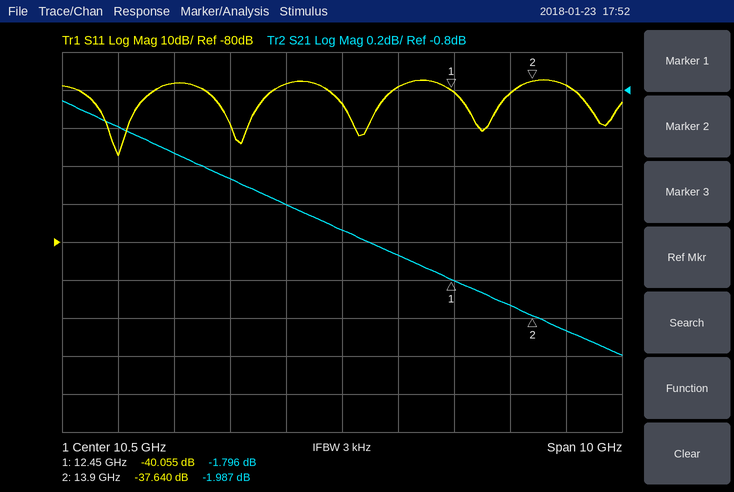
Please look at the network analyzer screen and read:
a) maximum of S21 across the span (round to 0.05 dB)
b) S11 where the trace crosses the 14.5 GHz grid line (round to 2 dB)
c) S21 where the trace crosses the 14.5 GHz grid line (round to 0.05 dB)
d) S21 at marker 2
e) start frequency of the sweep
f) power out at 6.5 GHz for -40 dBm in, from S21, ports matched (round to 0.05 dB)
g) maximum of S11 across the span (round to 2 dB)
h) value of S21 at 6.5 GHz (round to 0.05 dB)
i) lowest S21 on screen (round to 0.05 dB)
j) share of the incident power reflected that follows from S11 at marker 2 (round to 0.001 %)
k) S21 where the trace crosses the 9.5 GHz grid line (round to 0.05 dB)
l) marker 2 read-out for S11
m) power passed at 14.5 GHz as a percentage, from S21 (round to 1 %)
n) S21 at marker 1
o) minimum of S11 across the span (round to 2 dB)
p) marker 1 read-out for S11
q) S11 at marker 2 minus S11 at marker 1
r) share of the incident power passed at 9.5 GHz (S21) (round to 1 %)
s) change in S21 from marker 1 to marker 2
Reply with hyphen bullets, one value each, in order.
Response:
- -0.85 dB
- -38 dB
- -2.05 dB
- -1.987 dB
- 5.5 GHz
- -41.00 dBm
- -38 dB
- -1.00 dB
- -2.20 dB
- 0.017 %
- -1.40 dB
- -37.640 dB
- 62 %
- -1.796 dB
- -58 dB
- -40.055 dB
- 2.415 dB
- 72 %
- -0.191 dB
